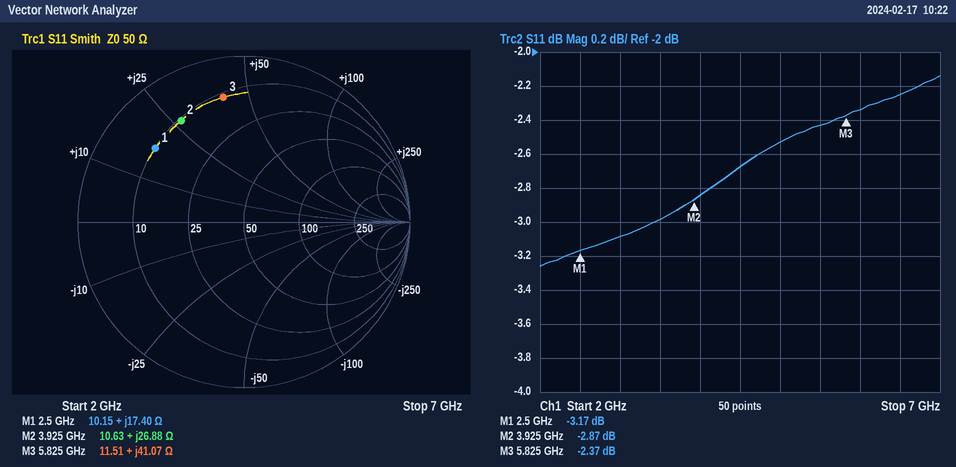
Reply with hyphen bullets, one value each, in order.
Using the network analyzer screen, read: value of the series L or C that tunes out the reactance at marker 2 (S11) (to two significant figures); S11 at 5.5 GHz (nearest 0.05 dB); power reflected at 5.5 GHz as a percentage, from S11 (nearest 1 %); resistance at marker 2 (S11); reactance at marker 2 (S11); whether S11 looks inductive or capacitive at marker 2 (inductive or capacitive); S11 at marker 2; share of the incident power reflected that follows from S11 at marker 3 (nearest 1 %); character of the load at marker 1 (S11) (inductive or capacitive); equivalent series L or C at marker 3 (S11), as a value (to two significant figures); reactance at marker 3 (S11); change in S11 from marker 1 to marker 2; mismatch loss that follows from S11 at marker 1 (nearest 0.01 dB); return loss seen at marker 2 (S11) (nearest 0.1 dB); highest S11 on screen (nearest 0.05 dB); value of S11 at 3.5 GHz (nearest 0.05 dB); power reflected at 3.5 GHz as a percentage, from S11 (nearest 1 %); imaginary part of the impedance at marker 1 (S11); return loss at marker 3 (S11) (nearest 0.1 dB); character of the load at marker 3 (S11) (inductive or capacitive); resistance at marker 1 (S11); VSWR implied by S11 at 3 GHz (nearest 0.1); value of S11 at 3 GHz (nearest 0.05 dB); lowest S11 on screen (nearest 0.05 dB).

- 1.5 pF
- -2.45 dB
- 57 %
- 10.63 Ω
- +26.88 Ω
- inductive
- -2.87 dB
- 58 %
- inductive
- 1.1 nH
- +41.07 Ω
- 0.30 dB
- 2.86 dB
- 2.9 dB
- -2.15 dB
- -3.00 dB
- 50 %
- +17.40 Ω
- 2.4 dB
- inductive
- 10.15 Ω
- 5.7
- -3.10 dB
- -3.25 dB
